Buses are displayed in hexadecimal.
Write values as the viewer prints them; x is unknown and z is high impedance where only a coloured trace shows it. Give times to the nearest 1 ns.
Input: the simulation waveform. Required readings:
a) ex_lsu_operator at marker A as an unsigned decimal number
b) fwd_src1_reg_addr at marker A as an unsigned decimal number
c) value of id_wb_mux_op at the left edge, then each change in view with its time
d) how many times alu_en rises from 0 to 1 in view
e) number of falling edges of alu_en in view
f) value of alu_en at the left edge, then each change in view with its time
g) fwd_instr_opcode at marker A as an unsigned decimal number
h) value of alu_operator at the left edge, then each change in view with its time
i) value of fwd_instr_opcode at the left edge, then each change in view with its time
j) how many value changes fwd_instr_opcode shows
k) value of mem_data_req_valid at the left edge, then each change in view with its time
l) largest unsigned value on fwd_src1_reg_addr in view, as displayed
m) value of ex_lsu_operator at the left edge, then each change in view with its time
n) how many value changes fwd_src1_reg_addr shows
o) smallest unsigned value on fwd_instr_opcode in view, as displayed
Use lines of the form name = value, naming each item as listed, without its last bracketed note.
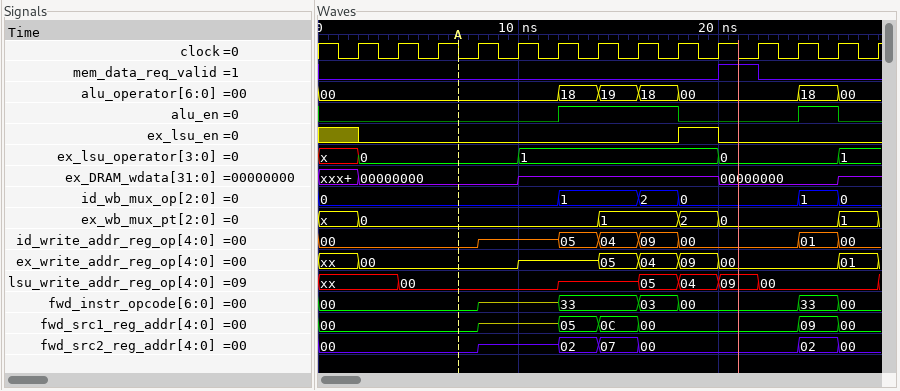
ex_lsu_operator at marker A as an unsigned decimal number = 0
fwd_src1_reg_addr at marker A as an unsigned decimal number = 0
value of id_wb_mux_op at the left edge, then each change in view with its time = 0, 1 at 12 ns, 2 at 16 ns, 0 at 18 ns, 1 at 24 ns, 0 at 26 ns
how many times alu_en rises from 0 to 1 in view = 2
number of falling edges of alu_en in view = 2
value of alu_en at the left edge, then each change in view with its time = 0, 1 at 12 ns, 0 at 18 ns, 1 at 24 ns, 0 at 26 ns
fwd_instr_opcode at marker A as an unsigned decimal number = 0
value of alu_operator at the left edge, then each change in view with its time = 00, 18 at 12 ns, 19 at 14 ns, 18 at 16 ns, 00 at 18 ns, 18 at 24 ns, 00 at 26 ns
value of fwd_instr_opcode at the left edge, then each change in view with its time = 00, z at 8 ns, 33 at 12 ns, 03 at 16 ns, 00 at 18 ns, 33 at 24 ns, 00 at 26 ns
how many value changes fwd_instr_opcode shows = 6
value of mem_data_req_valid at the left edge, then each change in view with its time = 0, 1 at 20 ns, 0 at 22 ns
largest unsigned value on fwd_src1_reg_addr in view, as displayed = 0C
value of ex_lsu_operator at the left edge, then each change in view with its time = x, 0 at 2 ns, 1 at 10 ns, 0 at 20 ns, 1 at 26 ns
how many value changes fwd_src1_reg_addr shows = 6
smallest unsigned value on fwd_instr_opcode in view, as displayed = 00
